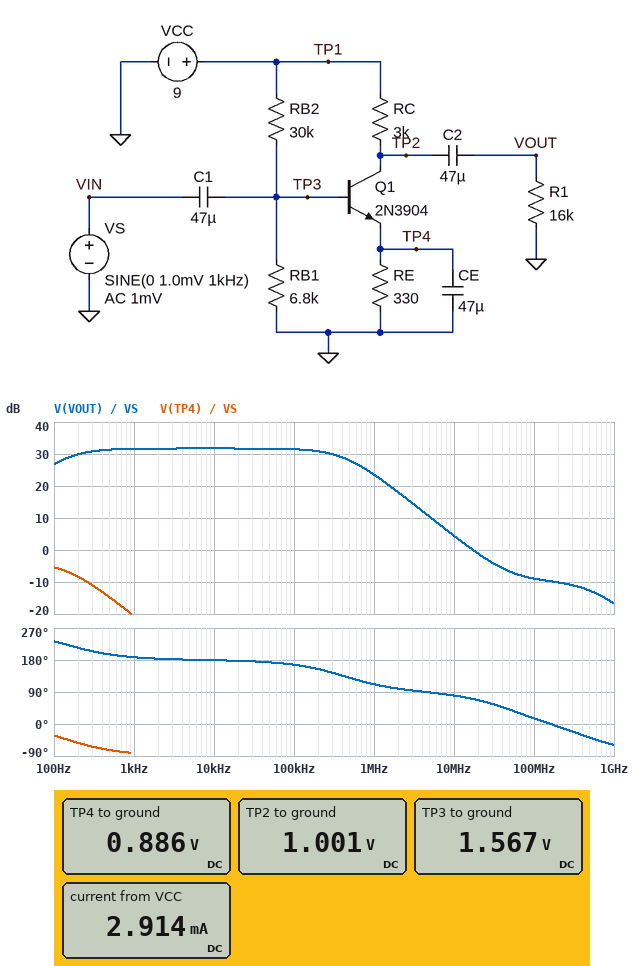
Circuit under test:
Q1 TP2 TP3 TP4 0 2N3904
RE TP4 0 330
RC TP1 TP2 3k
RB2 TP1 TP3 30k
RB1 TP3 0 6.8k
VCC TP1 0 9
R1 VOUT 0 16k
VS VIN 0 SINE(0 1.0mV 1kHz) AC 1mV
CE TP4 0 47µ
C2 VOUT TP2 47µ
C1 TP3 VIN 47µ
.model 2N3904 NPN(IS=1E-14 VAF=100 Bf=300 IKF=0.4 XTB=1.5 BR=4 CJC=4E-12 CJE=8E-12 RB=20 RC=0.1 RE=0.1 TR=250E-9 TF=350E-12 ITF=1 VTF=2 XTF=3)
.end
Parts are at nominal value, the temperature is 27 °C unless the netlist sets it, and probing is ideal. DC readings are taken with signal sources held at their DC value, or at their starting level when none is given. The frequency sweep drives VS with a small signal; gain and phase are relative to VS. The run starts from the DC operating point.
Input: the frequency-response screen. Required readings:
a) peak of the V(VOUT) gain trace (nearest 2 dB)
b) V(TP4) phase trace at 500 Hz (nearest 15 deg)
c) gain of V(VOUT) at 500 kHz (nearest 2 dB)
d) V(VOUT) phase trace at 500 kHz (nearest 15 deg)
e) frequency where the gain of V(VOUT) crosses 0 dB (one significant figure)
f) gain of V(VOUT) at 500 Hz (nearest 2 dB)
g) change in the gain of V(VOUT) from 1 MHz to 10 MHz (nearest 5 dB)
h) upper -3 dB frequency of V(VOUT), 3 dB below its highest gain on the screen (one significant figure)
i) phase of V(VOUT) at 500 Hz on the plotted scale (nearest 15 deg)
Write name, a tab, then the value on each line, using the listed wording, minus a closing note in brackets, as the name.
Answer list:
peak of the V(VOUT) gain trace	32 dB
V(TP4) phase trace at 500 Hz	-75 deg
gain of V(VOUT) at 500 kHz	28 dB
V(VOUT) phase trace at 500 kHz	135 deg
frequency where the gain of V(VOUT) crosses 0 dB	20 MHz
gain of V(VOUT) at 500 Hz	32 dB
change in the gain of V(VOUT) from 1 MHz to 10 MHz	-20 dB
upper -3 dB frequency of V(VOUT), 3 dB below its highest gain on the screen	400 kHz
phase of V(VOUT) at 500 Hz on the plotted scale	195 deg
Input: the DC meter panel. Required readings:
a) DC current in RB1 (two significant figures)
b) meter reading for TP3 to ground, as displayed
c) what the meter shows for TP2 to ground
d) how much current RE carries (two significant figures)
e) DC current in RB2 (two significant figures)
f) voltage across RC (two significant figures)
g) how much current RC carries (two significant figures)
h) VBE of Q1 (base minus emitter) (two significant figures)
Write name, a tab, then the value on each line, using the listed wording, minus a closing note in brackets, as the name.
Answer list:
DC current in RB1	230 µA
meter reading for TP3 to ground, as displayed	1.567 V
what the meter shows for TP2 to ground	1.001 V
how much current RE carries	2.7 mA
DC current in RB2	250 µA
voltage across RC	8.0 V
how much current RC carries	2.7 mA
VBE of Q1 (base minus emitter)	680 mV
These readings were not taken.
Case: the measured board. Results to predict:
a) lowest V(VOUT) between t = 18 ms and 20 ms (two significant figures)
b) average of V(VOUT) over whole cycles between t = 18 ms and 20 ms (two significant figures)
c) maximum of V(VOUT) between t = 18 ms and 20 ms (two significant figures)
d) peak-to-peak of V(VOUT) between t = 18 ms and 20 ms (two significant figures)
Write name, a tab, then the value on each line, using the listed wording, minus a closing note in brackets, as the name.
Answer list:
lowest V(VOUT) between t = 18 ms and 20 ms	-26 mV
average of V(VOUT) over whole cycles between t = 18 ms and 20 ms	14 mV
maximum of V(VOUT) between t = 18 ms and 20 ms	93 mV
peak-to-peak of V(VOUT) between t = 18 ms and 20 ms	120 mV
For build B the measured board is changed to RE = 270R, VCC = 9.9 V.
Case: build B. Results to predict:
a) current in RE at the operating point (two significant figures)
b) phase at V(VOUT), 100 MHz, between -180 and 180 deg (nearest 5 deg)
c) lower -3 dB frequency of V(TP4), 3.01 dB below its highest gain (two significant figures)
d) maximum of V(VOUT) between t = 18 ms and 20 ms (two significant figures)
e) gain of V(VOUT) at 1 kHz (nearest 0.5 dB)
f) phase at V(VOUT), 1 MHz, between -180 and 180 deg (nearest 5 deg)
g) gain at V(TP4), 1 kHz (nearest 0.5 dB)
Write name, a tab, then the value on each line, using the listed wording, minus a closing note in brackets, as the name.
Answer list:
current in RE at the operating point	3.1 mA
phase at V(VOUT), 100 MHz, between -180 and 180 deg	-5 deg
lower -3 dB frequency of V(TP4), 3.01 dB below its highest gain	5.8 Hz
maximum of V(VOUT) between t = 18 ms and 20 ms	10 mV
gain of V(VOUT) at 1 kHz	18.5 dB
phase at V(VOUT), 1 MHz, between -180 and 180 deg	105 deg
gain at V(TP4), 1 kHz	-23.5 dB
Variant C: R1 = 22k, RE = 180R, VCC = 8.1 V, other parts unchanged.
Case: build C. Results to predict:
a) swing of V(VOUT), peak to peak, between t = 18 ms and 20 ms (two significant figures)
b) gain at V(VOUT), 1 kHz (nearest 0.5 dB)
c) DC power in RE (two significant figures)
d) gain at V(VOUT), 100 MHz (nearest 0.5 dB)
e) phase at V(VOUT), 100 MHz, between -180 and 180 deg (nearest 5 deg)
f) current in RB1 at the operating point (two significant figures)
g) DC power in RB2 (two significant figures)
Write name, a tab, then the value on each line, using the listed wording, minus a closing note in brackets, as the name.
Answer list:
swing of V(VOUT), peak to peak, between t = 18 ms and 20 ms	13 mV
gain at V(VOUT), 1 kHz	16.0 dB
DC power in RE	1.2 mW
gain at V(VOUT), 100 MHz	-10.0 dB
phase at V(VOUT), 100 MHz, between -180 and 180 deg	-5 deg
current in RB1 at the operating point	170 µA
DC power in RB2	1.6 mW
